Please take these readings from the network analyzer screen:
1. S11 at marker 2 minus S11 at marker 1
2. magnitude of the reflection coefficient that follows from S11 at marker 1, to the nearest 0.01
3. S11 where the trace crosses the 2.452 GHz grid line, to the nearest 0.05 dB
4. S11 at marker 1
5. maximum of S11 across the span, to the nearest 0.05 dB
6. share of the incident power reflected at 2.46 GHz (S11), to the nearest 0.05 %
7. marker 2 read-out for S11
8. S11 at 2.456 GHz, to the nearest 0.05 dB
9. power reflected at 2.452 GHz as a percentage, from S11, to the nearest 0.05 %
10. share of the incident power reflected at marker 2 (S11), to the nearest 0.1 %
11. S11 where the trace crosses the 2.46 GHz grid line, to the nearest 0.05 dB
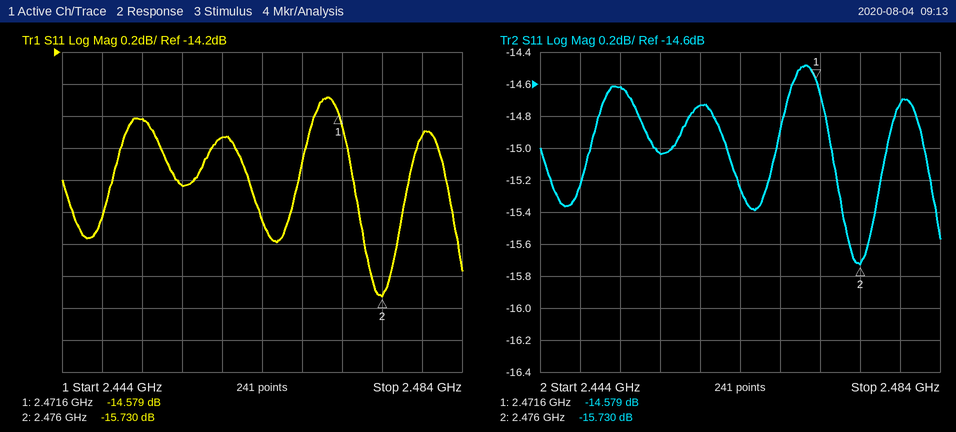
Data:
-1.151 dB
0.19
-14.60 dB
-14.579 dB
-14.50 dB
3.35 %
-15.730 dB
-15.05 dB
3.45 %
2.7 %
-14.75 dB
